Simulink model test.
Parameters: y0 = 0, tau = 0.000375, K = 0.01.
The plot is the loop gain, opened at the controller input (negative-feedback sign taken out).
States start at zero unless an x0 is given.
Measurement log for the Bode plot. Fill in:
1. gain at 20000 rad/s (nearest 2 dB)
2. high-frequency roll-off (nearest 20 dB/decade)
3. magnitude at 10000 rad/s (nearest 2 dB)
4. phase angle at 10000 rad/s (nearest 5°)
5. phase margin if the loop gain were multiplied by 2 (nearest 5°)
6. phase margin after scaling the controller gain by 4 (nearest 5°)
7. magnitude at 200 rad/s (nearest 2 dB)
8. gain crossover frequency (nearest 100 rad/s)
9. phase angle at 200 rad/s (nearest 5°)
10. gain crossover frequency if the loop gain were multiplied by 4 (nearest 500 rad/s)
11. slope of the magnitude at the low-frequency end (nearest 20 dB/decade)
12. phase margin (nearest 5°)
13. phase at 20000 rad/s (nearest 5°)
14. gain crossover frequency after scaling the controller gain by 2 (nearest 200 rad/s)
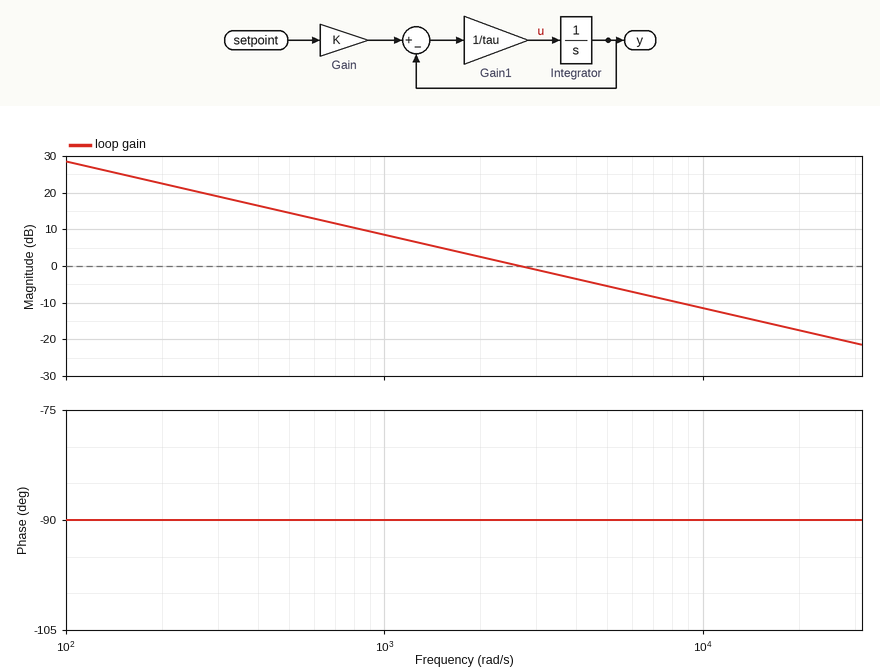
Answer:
-18 dB
-20 dB/decade
-12 dB
-90°
90°
90°
22 dB
2700 rad/s
-90°
10500 rad/s
-20 dB/decade
90°
-90°
5400 rad/s
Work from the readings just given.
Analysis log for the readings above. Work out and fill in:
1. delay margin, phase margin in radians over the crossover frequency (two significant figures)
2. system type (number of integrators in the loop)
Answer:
0.00058 s
1
